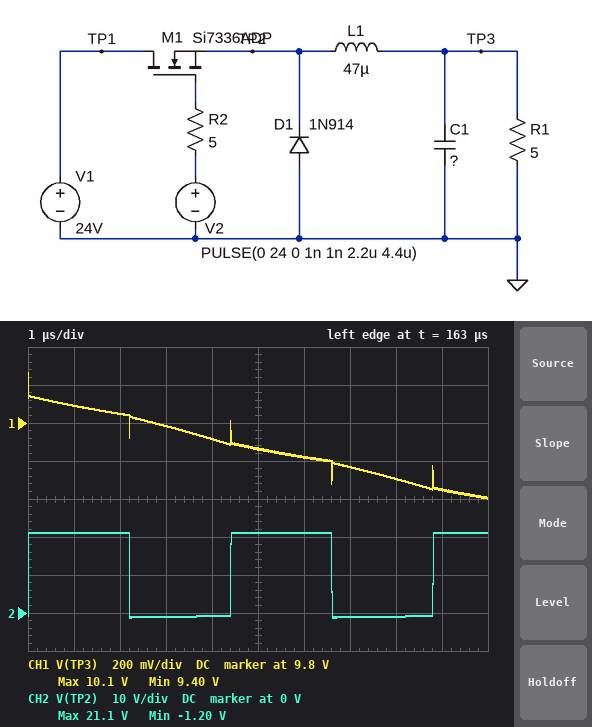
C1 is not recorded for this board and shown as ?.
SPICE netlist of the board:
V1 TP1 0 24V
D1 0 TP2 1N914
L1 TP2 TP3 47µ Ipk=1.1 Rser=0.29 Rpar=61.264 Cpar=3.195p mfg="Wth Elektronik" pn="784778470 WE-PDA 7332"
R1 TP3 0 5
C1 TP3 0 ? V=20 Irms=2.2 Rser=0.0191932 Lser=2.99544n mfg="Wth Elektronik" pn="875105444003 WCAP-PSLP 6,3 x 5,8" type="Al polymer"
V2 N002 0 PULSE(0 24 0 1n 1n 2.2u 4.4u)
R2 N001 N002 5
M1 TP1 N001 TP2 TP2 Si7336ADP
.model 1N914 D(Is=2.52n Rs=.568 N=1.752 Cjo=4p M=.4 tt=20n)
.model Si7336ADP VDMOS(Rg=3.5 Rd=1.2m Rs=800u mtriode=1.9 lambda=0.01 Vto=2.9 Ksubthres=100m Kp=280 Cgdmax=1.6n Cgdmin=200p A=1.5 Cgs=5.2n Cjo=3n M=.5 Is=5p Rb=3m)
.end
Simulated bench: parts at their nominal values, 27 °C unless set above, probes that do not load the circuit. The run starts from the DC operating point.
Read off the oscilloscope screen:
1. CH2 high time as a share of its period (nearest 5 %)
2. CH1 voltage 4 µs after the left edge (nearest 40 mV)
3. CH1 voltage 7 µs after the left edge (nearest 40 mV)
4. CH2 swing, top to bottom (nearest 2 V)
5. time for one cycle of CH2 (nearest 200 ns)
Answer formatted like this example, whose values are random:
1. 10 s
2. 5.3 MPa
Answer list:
1. 50 %
2. 9.72 V
3. 9.56 V
4. 22 V
5. 4.4 µs
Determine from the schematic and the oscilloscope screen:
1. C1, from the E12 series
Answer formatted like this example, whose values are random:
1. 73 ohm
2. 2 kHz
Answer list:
1. 27 µF
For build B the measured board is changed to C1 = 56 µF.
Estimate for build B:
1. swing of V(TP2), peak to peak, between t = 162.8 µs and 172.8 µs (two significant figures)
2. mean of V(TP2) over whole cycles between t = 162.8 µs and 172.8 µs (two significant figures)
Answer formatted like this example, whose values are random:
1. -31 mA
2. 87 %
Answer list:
1. 23 V
2. 9.6 V
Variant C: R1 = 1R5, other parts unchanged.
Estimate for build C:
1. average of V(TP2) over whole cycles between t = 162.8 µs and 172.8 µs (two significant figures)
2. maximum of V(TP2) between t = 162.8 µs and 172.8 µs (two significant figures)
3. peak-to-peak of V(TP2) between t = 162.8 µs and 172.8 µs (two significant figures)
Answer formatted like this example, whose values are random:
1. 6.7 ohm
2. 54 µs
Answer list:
1. 9.0 V
2. 21 V
3. 24 V
